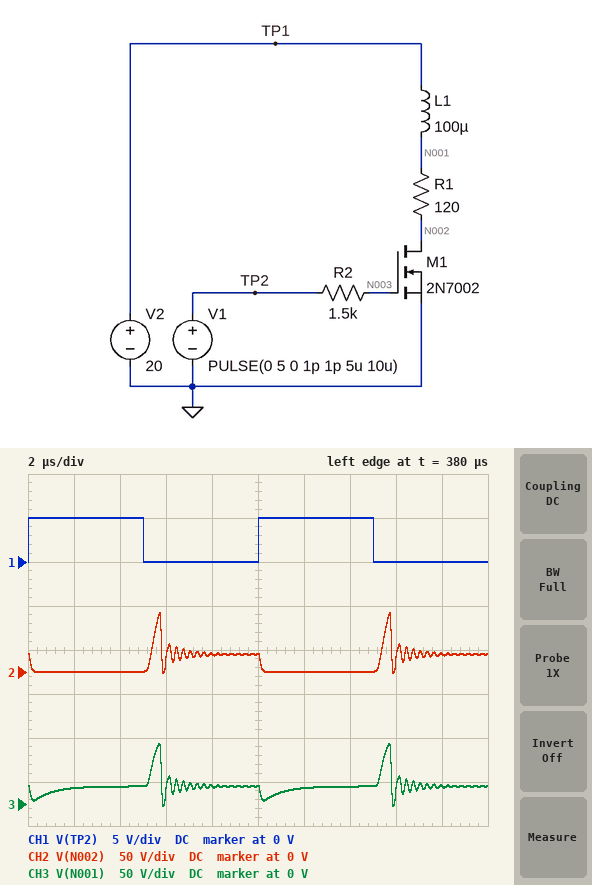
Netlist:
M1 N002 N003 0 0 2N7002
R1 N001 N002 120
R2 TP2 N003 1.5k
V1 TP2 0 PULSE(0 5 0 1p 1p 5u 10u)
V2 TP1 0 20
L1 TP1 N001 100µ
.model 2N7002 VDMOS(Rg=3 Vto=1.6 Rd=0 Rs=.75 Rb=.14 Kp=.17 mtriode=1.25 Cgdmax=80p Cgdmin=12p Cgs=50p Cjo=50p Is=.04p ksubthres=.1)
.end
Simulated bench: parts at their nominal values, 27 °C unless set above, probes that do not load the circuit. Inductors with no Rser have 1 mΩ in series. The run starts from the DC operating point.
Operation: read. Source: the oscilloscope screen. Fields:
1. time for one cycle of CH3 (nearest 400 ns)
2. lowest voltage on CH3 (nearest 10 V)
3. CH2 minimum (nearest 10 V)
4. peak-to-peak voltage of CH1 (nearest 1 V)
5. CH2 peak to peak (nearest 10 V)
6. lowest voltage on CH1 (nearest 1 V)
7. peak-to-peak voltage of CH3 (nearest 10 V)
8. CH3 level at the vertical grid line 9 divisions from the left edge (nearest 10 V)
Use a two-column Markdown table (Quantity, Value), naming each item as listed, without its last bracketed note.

| Quantity | Value |
|---|---|
| time for one cycle of CH3 | 10.0 µs |
| lowest voltage on CH3 | 0 V |
| CH2 minimum | 0 V |
| peak-to-peak voltage of CH1 | 5 V |
| CH2 peak to peak | 70 V |
| lowest voltage on CH1 | 0 V |
| peak-to-peak voltage of CH3 | 70 V |
| CH3 level at the vertical grid line 9 divisions from the left edge | 20 V |
